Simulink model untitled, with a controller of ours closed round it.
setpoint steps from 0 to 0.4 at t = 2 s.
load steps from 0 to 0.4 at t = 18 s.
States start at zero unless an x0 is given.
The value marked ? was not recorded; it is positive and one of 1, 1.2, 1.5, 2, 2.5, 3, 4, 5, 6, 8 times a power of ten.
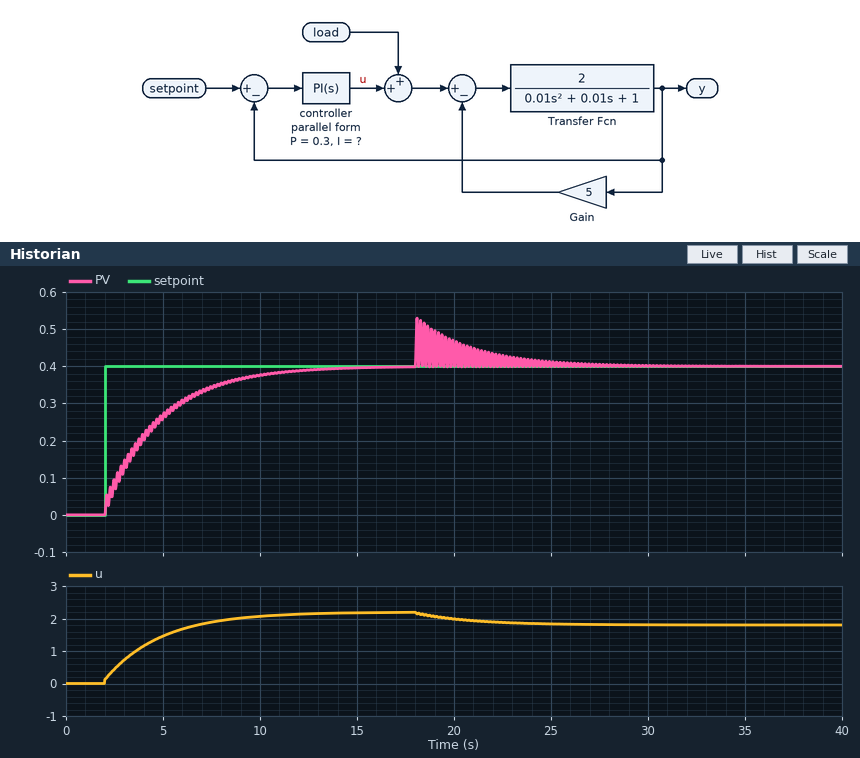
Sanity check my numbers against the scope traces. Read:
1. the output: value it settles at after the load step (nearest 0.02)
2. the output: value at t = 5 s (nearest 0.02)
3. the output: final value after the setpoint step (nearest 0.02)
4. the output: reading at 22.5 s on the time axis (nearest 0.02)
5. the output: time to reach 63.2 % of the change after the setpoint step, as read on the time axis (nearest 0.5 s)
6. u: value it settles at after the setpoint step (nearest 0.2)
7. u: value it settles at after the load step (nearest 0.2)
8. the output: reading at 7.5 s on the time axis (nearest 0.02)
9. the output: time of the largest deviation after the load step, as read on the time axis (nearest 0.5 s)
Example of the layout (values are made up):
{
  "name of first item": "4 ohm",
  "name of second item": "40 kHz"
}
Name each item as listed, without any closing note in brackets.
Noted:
{
  "the output: value it settles at after the load step": "0.40",
  "the output: value at t = 5 s": "0.26",
  "the output: final value after the setpoint step": "0.40",
  "the output: reading at 22.5 s on the time axis": "0.42",
  "the output: time to reach 63.2 % of the change after the setpoint step, as read on the time axis": "4.5 s",
  "u: value it settles at after the setpoint step": "2.2",
  "u: value it settles at after the load step": "1.8",
  "the output: reading at 7.5 s on the time axis": "0.34",
  "the output: time of the largest deviation after the load step, as read on the time axis": "18.0 s"
}
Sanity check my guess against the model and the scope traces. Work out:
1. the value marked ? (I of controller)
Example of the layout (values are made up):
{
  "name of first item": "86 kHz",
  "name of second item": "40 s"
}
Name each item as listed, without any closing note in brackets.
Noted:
{
  "the value marked ?": "2"
}
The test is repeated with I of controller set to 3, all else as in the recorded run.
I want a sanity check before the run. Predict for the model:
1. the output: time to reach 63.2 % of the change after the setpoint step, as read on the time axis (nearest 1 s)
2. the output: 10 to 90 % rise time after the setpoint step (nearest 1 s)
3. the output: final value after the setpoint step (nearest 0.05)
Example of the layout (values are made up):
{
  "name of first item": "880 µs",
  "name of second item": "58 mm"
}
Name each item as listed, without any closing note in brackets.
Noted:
{
  "the output: time to reach 63.2 % of the change after the setpoint step, as read on the time axis": "4 s",
  "the output: 10 to 90 % rise time after the setpoint step": "4 s",
  "the output: final value after the setpoint step": "0.40"
}
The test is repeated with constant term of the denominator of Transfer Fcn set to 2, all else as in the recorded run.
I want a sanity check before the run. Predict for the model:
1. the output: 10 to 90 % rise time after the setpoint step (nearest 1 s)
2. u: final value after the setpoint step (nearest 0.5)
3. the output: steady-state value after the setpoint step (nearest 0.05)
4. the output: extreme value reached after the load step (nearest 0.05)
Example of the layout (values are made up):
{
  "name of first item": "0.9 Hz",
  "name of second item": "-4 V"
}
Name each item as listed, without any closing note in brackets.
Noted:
{
  "the output: 10 to 90 % rise time after the setpoint step": "7 s",
  "u: final value after the setpoint step": "2.5",
  "the output: steady-state value after the setpoint step": "0.40",
  "the output: extreme value reached after the load step": "0.50"
}
